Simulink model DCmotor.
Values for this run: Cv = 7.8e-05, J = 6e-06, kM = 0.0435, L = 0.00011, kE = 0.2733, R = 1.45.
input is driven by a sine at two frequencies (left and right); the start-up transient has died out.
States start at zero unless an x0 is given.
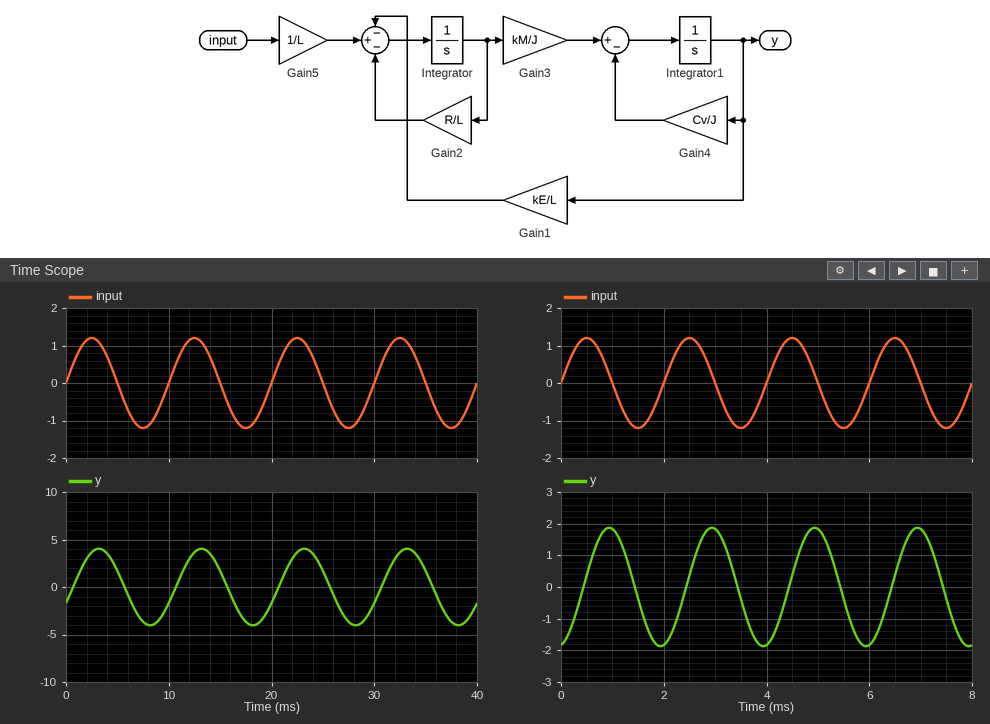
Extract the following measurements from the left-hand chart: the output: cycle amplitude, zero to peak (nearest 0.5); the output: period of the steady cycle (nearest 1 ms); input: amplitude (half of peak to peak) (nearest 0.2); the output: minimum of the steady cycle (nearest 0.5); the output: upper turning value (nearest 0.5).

4.0
10 ms
1.2
-4.0
4.0
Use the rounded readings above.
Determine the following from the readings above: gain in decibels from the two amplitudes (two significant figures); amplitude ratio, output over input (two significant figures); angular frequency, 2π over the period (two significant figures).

10 dB
3.3
0.63 rad/ms
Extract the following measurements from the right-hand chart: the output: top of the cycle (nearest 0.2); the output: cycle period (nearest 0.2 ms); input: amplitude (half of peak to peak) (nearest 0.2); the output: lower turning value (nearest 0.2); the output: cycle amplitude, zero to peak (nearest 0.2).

1.8
2.0 ms
1.2
-1.8
1.8
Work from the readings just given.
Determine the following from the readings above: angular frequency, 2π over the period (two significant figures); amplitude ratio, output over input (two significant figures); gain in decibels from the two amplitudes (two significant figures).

3.1 rad/ms
1.5
3.5 dB
